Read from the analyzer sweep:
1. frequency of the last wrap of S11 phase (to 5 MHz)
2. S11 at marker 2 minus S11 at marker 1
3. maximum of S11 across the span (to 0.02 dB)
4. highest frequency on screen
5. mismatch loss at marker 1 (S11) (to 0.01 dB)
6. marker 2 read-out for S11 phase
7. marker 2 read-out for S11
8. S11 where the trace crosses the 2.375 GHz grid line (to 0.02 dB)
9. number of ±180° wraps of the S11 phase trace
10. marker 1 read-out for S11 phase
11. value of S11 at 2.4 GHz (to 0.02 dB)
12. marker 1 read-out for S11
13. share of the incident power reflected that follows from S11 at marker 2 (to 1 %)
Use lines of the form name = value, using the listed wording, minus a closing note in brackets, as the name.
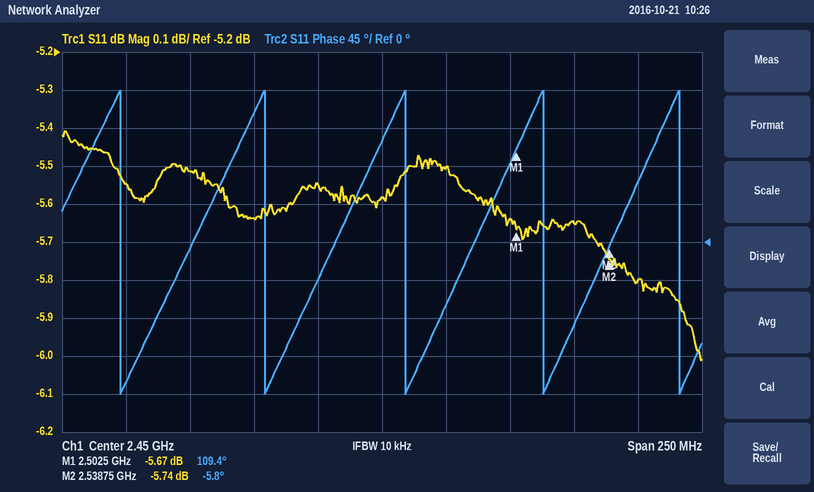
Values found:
frequency of the last wrap of S11 phase = 2.565 GHz
S11 at marker 2 minus S11 at marker 1 = -0.07 dB
maximum of S11 across the span = -5.40 dB
highest frequency on screen = 2.575 GHz
mismatch loss at marker 1 (S11) = 1.37 dB
marker 2 read-out for S11 phase = -5.8°
marker 2 read-out for S11 = -5.74 dB
S11 where the trace crosses the 2.375 GHz grid line = -5.52 dB
number of ±180° wraps of the S11 phase trace = 5
marker 1 read-out for S11 phase = 109.4°
value of S11 at 2.4 GHz = -5.64 dB
marker 1 read-out for S11 = -5.67 dB
share of the incident power reflected that follows from S11 at marker 2 = 27 %
